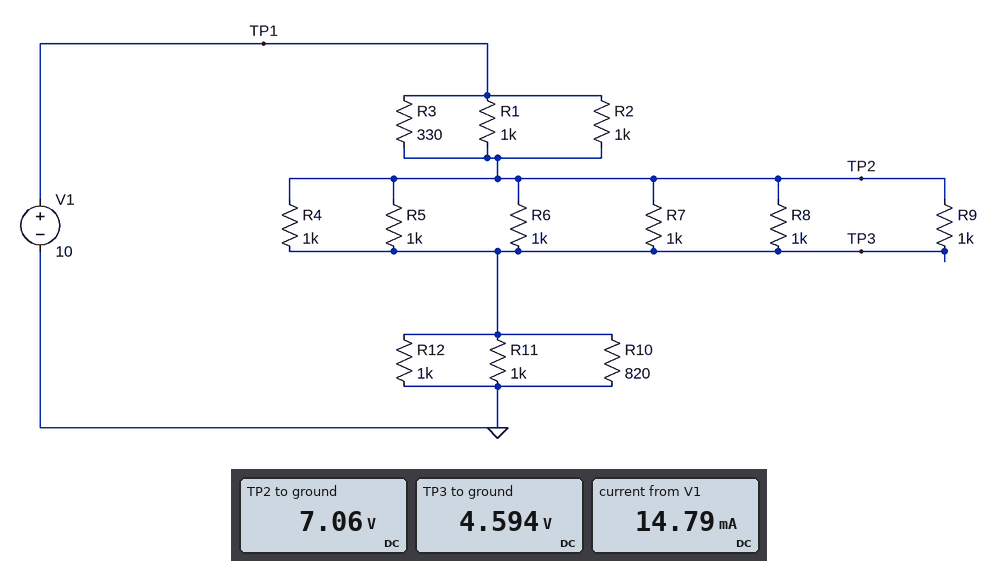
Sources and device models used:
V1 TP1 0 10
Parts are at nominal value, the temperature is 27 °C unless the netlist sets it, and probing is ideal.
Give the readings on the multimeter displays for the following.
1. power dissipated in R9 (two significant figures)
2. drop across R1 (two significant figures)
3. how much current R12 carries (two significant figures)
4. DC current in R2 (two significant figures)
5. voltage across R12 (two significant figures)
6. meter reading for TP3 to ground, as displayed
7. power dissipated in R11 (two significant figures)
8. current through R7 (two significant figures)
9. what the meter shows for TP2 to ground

6.1 mW
2.9 V
4.6 mA
2.9 mA
4.6 V
4.594 V
21 mW
2.5 mA
7.06 V
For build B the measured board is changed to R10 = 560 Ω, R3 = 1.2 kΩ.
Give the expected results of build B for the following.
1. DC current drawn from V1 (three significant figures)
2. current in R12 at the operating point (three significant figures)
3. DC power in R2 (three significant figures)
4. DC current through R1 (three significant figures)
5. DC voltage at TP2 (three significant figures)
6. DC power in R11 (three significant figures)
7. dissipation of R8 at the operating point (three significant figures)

12.8 mA
3.37 mA
20.3 mW
4.50 mA
5.50 V
11.4 mW
4.52 mW
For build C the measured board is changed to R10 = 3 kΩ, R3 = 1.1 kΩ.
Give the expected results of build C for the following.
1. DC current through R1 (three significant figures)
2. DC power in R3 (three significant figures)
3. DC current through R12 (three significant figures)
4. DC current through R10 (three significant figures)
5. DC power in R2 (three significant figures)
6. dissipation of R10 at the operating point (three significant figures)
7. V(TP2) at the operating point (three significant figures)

3.66 mA
12.2 mW
4.56 mA
1.52 mA
13.4 mW
6.94 mW
6.34 V
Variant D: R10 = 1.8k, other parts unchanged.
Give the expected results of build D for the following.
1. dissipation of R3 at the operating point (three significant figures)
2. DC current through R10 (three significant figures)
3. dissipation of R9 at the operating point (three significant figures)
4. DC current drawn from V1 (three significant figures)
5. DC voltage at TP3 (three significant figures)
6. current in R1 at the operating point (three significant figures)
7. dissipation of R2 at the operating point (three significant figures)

20.9 mW
2.87 mA
4.85 mW
13.2 mA
5.17 V
2.63 mA
6.90 mW
